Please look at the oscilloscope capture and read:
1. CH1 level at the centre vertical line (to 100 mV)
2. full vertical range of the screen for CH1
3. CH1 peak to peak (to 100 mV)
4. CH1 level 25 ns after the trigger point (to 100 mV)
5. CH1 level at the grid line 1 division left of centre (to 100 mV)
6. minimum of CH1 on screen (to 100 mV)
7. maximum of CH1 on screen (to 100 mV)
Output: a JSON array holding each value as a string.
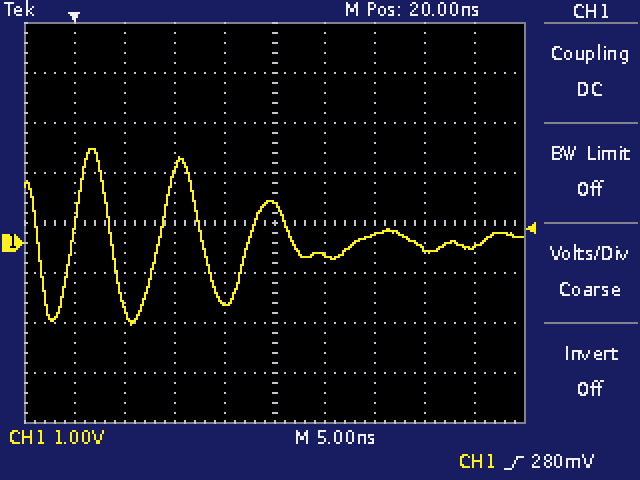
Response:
["800 mV", "8 V", "3.5 V", "-200 mV", "-1.2 V", "-1.6 V", "1.9 V"]
